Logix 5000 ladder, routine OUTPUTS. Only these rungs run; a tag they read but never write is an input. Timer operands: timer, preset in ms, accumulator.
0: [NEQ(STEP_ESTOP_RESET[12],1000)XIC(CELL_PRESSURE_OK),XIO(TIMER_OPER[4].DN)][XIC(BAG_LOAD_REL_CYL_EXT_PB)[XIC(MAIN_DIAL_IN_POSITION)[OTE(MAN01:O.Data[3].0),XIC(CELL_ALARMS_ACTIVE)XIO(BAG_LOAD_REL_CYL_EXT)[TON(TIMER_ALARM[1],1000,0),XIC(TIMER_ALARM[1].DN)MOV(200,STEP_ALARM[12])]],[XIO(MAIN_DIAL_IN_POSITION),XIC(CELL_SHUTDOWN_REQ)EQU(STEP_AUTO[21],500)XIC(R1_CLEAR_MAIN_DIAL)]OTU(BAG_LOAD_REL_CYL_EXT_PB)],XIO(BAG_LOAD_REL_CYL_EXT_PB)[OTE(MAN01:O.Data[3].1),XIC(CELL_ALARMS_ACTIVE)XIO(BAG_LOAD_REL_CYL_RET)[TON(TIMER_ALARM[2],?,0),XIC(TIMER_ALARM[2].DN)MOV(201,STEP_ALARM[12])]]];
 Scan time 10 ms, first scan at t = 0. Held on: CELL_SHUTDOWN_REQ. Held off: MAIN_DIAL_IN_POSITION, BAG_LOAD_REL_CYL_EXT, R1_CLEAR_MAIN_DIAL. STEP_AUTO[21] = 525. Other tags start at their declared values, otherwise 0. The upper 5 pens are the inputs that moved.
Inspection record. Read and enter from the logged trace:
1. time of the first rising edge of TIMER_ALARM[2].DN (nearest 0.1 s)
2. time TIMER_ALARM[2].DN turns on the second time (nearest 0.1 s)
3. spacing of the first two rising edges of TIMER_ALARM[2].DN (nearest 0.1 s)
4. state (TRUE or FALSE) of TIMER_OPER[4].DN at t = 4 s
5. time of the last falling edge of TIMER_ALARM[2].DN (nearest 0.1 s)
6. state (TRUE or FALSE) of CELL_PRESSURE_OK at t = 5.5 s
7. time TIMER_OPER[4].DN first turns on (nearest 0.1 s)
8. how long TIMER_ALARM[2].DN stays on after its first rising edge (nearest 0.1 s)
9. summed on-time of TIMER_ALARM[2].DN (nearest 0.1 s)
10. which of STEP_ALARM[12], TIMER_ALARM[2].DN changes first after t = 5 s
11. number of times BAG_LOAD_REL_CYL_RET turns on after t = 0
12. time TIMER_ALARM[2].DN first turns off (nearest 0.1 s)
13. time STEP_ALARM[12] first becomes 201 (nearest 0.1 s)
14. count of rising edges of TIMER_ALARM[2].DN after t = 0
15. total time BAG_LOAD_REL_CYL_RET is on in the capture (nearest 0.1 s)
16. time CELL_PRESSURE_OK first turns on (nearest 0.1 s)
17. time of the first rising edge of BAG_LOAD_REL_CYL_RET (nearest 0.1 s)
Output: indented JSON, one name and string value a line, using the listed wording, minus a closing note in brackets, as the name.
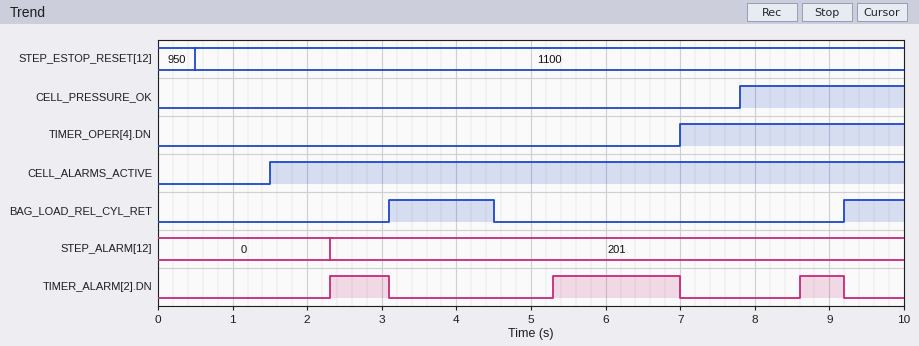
{
  "time of the first rising edge of TIMER_ALARM[2].DN": "2.3 s",
  "time TIMER_ALARM[2].DN turns on the second time": "5.3 s",
  "spacing of the first two rising edges of TIMER_ALARM[2].DN": "3.0 s",
  "state (TRUE or FALSE) of TIMER_OPER[4].DN at t = 4 s": "FALSE",
  "time of the last falling edge of TIMER_ALARM[2].DN": "9.2 s",
  "state (TRUE or FALSE) of CELL_PRESSURE_OK at t = 5.5 s": "FALSE",
  "time TIMER_OPER[4].DN first turns on": "7.0 s",
  "how long TIMER_ALARM[2].DN stays on after its first rising edge": "0.8 s",
  "summed on-time of TIMER_ALARM[2].DN": "3.1 s",
  "which of STEP_ALARM[12], TIMER_ALARM[2].DN changes first after t = 5 s": "TIMER_ALARM[2].DN",
  "number of times BAG_LOAD_REL_CYL_RET turns on after t = 0": "2",
  "time TIMER_ALARM[2].DN first turns off": "3.1 s",
  "time STEP_ALARM[12] first becomes 201": "2.3 s",
  "count of rising edges of TIMER_ALARM[2].DN after t = 0": "3",
  "total time BAG_LOAD_REL_CYL_RET is on in the capture": "2.2 s",
  "time CELL_PRESSURE_OK first turns on": "7.8 s",
  "time of the first rising edge of BAG_LOAD_REL_CYL_RET": "3.1 s"
}
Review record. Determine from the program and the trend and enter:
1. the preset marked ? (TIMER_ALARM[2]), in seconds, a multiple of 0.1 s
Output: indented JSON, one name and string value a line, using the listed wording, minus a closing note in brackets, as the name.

{
  "the preset marked ? (TIMER_ALARM[2]), in seconds, a multiple of 0.1 s": "0.8 s"
}
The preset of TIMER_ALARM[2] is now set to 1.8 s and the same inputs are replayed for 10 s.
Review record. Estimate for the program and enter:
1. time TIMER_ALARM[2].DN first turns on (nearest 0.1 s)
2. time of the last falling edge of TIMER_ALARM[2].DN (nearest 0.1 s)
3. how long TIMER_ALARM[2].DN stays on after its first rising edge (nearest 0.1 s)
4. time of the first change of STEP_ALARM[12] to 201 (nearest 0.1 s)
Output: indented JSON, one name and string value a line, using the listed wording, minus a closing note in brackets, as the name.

{
  "time TIMER_ALARM[2].DN first turns on": "6.3 s",
  "time of the last falling edge of TIMER_ALARM[2].DN": "7.0 s",
  "how long TIMER_ALARM[2].DN stays on after its first rising edge": "0.7 s",
  "time of the first change of STEP_ALARM[12] to 201": "6.3 s"
}
